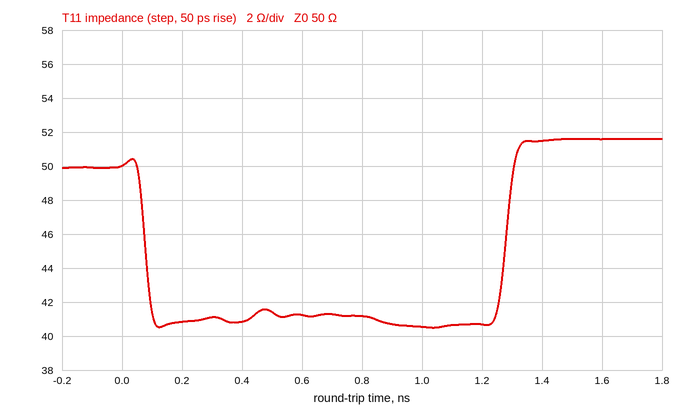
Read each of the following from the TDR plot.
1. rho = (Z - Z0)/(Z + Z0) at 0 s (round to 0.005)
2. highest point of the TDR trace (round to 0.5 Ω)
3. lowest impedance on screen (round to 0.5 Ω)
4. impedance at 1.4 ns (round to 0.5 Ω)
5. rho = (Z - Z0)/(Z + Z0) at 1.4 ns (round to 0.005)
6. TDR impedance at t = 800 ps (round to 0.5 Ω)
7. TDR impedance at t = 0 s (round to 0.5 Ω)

0.000
51.5 Ω
40.5 Ω
51.5 Ω
+0.015
41.0 Ω
50.0 Ω
